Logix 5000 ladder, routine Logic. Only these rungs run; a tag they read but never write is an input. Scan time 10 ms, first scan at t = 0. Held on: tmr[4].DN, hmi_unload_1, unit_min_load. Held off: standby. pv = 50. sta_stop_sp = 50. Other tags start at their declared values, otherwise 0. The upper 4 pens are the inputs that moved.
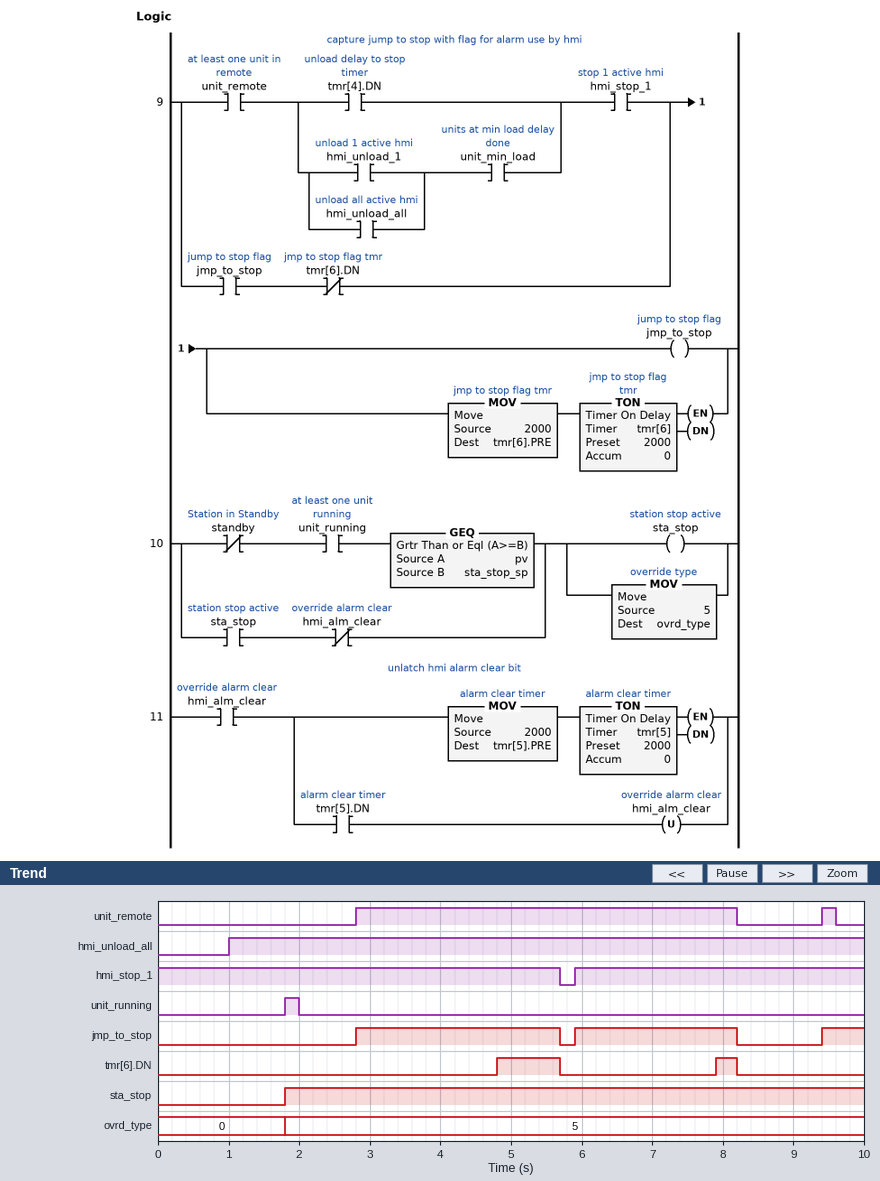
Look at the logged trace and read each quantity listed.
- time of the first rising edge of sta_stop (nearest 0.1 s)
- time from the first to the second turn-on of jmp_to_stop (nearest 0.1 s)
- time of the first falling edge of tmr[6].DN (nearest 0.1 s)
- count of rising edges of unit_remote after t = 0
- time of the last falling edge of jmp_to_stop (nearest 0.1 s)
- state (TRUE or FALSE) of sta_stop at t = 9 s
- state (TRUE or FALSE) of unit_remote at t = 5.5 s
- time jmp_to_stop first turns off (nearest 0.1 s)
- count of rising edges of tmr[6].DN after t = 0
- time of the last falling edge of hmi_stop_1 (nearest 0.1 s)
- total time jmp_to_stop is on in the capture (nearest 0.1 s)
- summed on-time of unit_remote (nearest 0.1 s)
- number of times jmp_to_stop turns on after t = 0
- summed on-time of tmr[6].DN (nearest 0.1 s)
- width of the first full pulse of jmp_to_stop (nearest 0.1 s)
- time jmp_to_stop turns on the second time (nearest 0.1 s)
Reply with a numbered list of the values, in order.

1. 1.8 s
2. 3.1 s
3. 5.7 s
4. 2
5. 8.2 s
6. TRUE
7. TRUE
8. 5.7 s
9. 2
10. 5.7 s
11. 5.8 s
12. 5.6 s
13. 3
14. 1.2 s
15. 2.9 s
16. 5.9 s
